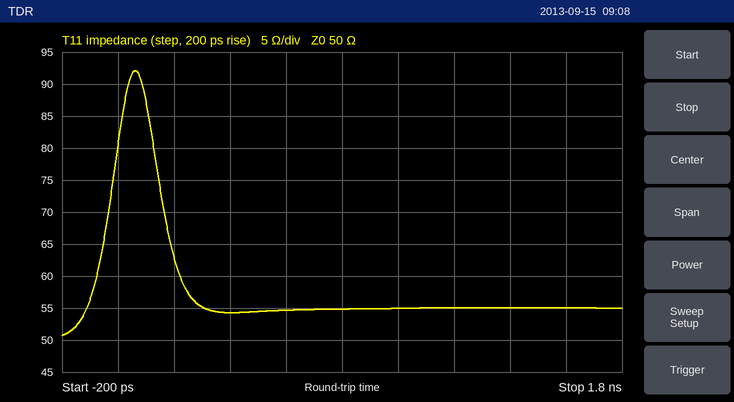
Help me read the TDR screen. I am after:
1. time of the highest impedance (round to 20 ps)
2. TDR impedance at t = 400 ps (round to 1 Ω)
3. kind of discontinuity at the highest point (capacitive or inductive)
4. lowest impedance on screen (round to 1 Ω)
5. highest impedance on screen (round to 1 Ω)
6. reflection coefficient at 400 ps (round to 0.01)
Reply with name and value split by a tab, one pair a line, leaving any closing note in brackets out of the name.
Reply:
time of the highest impedance	60 ps
TDR impedance at t = 400 ps	54 Ω
kind of discontinuity at the highest point	inductive
lowest impedance on screen	51 Ω
highest impedance on screen	92 Ω
reflection coefficient at 400 ps	+0.04
